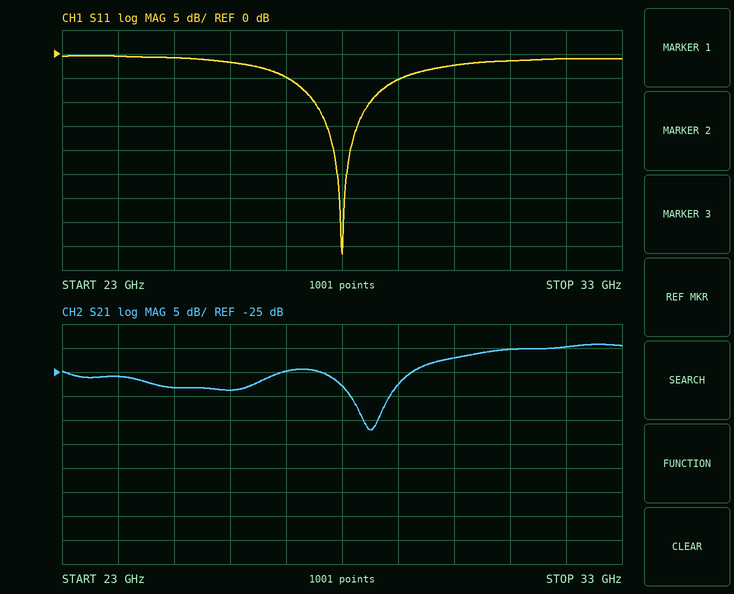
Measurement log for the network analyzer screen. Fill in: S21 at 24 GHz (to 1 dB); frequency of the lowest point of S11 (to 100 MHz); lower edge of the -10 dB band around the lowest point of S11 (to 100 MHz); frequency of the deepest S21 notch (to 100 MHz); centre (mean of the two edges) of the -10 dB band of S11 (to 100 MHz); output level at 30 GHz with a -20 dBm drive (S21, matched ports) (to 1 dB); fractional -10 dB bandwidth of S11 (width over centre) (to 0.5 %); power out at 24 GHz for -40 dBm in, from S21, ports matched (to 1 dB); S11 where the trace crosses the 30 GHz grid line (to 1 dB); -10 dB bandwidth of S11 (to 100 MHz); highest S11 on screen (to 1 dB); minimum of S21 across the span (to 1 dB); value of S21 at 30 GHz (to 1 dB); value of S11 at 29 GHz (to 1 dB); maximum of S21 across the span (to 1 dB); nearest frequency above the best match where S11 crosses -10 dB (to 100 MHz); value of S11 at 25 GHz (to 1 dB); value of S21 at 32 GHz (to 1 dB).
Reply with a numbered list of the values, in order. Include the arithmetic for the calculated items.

1. -26 dB
2. 28.0 GHz
3. 27.5 GHz
4. 28.5 GHz
5. 28.0 GHz
6. -20 dBm + (-22 dB) = -42 dBm
7. 1 GHz / 28 GHz ≈ 3.57 %, so 3.5 % to the nearest 0.5 %
8. -40 dBm + (-26 dB) = -66 dBm
9. -2 dB
10. 28.5 GHz − 27.5 GHz = 1.0 GHz
11. 0 dB
12. -37 dB
13. -22 dB
14. -5 dB
15. -19 dB
16. 28.5 GHz
17. -1 dB
18. -20 dB
